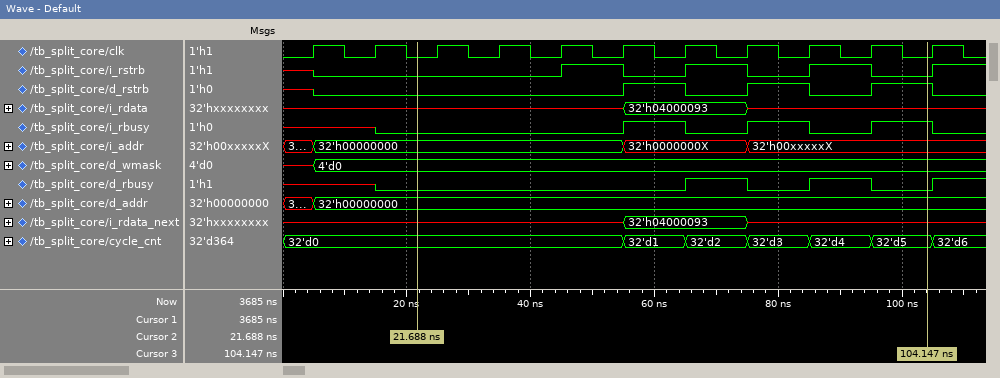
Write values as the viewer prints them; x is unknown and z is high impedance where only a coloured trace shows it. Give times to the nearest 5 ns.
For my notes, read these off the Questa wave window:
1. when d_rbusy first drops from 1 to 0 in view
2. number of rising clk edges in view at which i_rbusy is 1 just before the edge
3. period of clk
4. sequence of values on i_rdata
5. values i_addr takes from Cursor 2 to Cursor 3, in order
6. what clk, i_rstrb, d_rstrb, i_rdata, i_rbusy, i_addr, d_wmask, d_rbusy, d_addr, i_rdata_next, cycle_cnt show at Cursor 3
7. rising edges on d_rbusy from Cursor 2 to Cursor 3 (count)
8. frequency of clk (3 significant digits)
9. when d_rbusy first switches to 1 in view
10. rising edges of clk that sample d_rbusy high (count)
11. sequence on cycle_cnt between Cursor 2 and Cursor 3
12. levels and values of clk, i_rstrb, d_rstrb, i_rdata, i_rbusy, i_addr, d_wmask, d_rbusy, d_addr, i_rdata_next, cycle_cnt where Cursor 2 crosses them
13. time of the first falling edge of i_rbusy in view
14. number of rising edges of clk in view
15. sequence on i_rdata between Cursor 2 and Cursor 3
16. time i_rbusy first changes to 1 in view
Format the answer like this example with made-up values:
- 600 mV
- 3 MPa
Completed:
- 75 ns
- 3
- 10 ns
- x, 32'h04000093, x
- 32'h00000000, 32'h0000000X, 32'h00xxxxxX
- clk=0, i_rstrb=0, d_rstrb=1, i_rdata=x, i_rbusy=1, i_addr=32'h00xxxxxX, d_wmask=4'd0, d_rbusy=0, d_addr=32'h00000000, i_rdata_next=x, cycle_cnt=32'd5
- 2
- 100 MHz
- 65 ns
- 2
- 32'd0, 32'd1, 32'd2, 32'd3, 32'd4, 32'd5
- clk=0, i_rstrb=0, d_rstrb=0, i_rdata=x, i_rbusy=0, i_addr=32'h00000000, d_wmask=4'd0, d_rbusy=0, d_addr=32'h00000000, i_rdata_next=x, cycle_cnt=32'd0
- 65 ns
- 11
- x, 32'h04000093, x
- 55 ns
